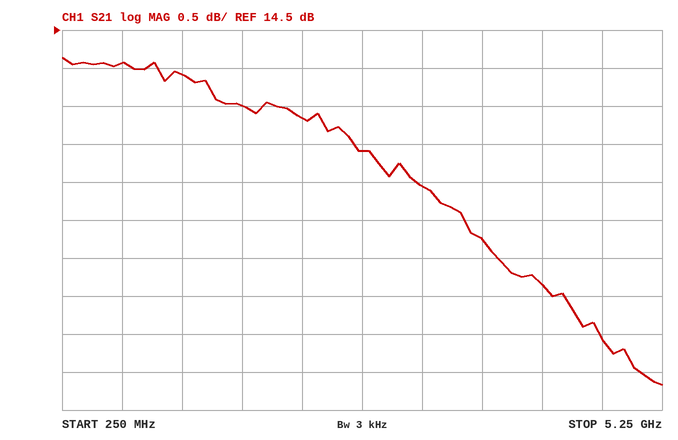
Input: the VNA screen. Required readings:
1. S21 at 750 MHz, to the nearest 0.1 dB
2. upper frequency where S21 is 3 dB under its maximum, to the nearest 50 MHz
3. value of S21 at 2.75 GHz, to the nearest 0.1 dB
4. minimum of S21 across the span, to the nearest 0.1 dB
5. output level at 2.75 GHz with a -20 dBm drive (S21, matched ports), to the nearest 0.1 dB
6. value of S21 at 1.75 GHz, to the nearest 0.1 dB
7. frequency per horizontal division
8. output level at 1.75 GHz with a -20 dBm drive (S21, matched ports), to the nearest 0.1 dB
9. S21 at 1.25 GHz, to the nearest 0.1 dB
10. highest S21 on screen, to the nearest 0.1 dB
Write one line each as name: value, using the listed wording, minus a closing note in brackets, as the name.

S21 at 750 MHz, to the nearest 0.1 dB: 14.1 dB
upper frequency where S21 is 3 dB under its maximum, to the nearest 50 MHz: 4.25 GHz
value of S21 at 2.75 GHz, to the nearest 0.1 dB: 12.9 dB
minimum of S21 across the span, to the nearest 0.1 dB: 9.8 dB
output level at 2.75 GHz with a -20 dBm drive (S21, matched ports), to the nearest 0.1 dB: -7.1 dBm
value of S21 at 1.75 GHz, to the nearest 0.1 dB: 13.5 dB
frequency per horizontal division: 500 MHz
output level at 1.75 GHz with a -20 dBm drive (S21, matched ports), to the nearest 0.1 dB: -6.5 dBm
S21 at 1.25 GHz, to the nearest 0.1 dB: 13.9 dB
highest S21 on screen, to the nearest 0.1 dB: 14.1 dB
